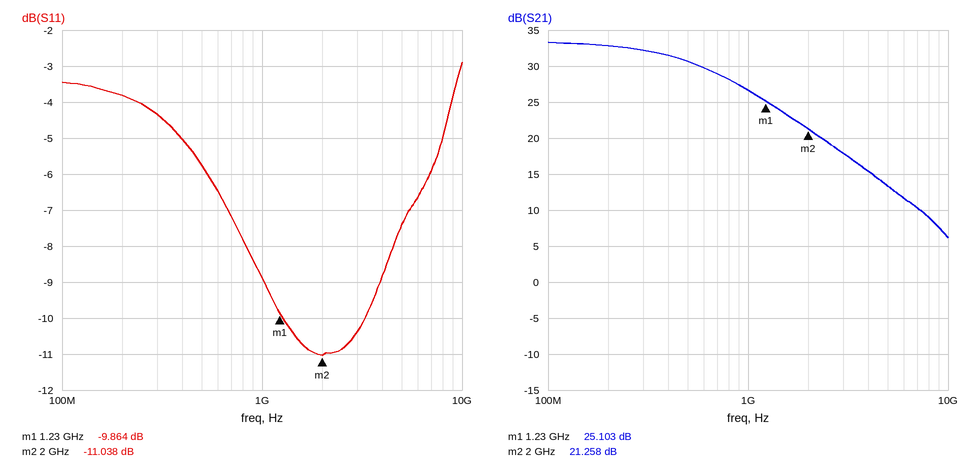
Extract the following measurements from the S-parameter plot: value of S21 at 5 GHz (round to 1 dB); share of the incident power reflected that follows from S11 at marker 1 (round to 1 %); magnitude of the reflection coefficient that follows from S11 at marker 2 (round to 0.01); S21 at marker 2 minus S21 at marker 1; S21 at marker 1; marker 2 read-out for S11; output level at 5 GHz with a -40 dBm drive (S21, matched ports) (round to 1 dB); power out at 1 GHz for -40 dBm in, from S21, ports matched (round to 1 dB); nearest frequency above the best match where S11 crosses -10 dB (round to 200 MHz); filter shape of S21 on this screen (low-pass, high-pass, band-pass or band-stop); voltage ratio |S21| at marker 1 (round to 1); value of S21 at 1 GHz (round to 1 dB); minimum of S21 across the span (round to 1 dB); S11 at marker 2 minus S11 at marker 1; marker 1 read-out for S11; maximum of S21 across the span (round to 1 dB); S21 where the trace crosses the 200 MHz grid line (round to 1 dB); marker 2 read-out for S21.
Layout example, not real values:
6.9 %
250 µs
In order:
13 dB
10 %
0.28
-3.845 dB
25.103 dB
-11.038 dB
-27 dBm
-13 dBm
3.2 GHz
low-pass
18
27 dB
6 dB
-1.174 dB
-9.864 dB
33 dB
33 dB
21.258 dB
